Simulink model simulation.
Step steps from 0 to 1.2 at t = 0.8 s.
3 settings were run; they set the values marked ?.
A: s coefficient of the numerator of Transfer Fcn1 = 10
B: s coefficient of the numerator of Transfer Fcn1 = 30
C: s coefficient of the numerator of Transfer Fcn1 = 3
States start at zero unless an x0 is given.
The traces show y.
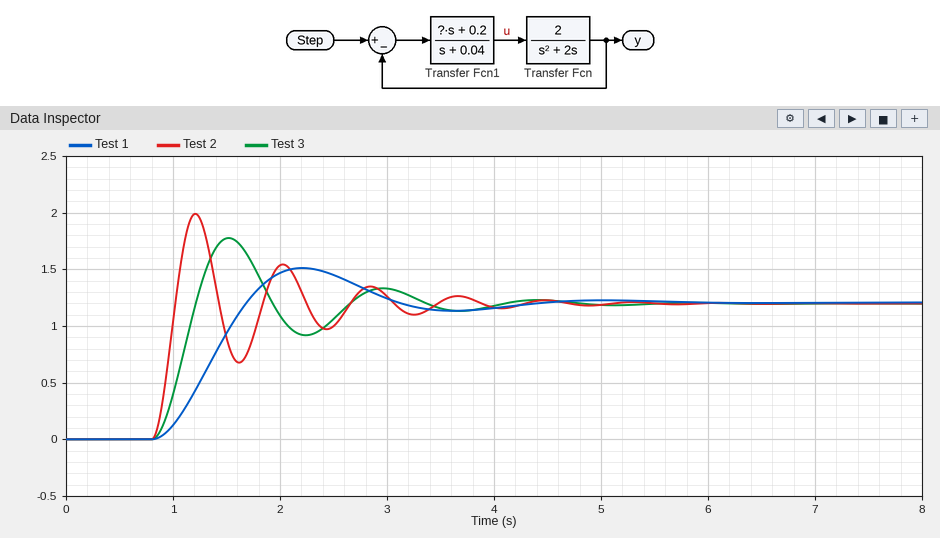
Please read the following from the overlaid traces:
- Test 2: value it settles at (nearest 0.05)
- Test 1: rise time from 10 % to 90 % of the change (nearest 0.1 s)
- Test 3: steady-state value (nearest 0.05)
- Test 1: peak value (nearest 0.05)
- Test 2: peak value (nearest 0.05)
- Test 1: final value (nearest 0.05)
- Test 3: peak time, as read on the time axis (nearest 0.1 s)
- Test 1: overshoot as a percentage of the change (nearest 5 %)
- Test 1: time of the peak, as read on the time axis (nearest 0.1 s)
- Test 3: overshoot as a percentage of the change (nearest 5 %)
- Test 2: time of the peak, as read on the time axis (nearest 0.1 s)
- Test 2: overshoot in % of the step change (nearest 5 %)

1.20
0.6 s
1.20
1.50
2.00
1.20
1.5 s
25 %
2.2 s
50 %
1.2 s
65 %
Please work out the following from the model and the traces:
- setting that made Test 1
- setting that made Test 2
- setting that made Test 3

C
B
A
